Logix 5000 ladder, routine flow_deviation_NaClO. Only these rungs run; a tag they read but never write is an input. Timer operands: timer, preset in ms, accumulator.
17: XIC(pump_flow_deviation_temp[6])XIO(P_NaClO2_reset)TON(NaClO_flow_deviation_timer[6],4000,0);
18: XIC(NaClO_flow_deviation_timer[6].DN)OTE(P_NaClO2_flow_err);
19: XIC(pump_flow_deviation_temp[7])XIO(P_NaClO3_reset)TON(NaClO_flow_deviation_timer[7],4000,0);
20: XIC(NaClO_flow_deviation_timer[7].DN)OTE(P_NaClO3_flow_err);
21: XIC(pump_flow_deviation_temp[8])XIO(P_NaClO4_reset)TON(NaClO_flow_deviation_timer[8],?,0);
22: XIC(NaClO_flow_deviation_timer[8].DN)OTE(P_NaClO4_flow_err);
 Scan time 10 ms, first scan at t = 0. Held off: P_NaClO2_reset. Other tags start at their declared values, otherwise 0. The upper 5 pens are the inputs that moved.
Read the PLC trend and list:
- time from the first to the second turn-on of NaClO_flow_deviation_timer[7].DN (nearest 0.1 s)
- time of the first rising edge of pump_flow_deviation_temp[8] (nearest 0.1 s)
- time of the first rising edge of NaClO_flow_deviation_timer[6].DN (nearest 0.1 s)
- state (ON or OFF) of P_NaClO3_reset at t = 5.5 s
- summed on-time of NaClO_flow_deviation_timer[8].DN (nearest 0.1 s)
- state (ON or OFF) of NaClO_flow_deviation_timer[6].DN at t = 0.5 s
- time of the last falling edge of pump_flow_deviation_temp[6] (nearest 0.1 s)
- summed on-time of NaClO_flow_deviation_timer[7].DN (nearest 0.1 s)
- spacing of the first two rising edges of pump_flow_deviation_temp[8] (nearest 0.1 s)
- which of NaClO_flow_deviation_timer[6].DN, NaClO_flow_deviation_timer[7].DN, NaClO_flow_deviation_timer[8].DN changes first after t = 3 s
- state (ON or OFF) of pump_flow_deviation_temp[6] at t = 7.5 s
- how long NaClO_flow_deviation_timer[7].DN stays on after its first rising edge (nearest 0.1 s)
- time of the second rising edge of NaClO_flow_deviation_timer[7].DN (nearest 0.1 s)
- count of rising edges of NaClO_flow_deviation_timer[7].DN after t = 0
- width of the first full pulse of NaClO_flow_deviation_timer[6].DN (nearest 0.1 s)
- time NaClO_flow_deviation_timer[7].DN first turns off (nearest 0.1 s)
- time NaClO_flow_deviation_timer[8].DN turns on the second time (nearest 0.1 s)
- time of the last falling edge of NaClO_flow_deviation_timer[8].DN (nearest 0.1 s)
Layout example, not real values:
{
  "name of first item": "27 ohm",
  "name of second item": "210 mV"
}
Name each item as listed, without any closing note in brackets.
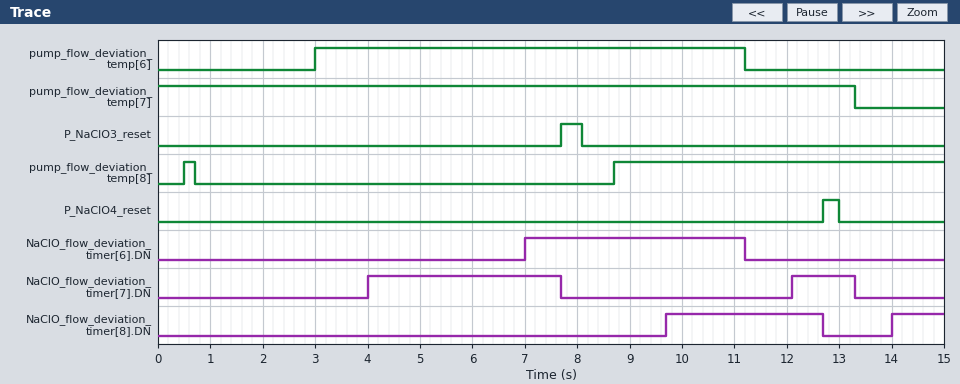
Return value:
{
  "time from the first to the second turn-on of NaClO_flow_deviation_timer[7].DN": "8.1 s",
  "time of the first rising edge of pump_flow_deviation_temp[8]": "0.5 s",
  "time of the first rising edge of NaClO_flow_deviation_timer[6].DN": "7.0 s",
  "state (ON or OFF) of P_NaClO3_reset at t = 5.5 s": "OFF",
  "summed on-time of NaClO_flow_deviation_timer[8].DN": "4.0 s",
  "state (ON or OFF) of NaClO_flow_deviation_timer[6].DN at t = 0.5 s": "OFF",
  "time of the last falling edge of pump_flow_deviation_temp[6]": "11.2 s",
  "summed on-time of NaClO_flow_deviation_timer[7].DN": "4.9 s",
  "spacing of the first two rising edges of pump_flow_deviation_temp[8]": "8.2 s",
  "which of NaClO_flow_deviation_timer[6].DN, NaClO_flow_deviation_timer[7].DN, NaClO_flow_deviation_timer[8].DN changes first after t = 3 s": "NaClO_flow_deviation_timer[7].DN",
  "state (ON or OFF) of pump_flow_deviation_temp[6] at t = 7.5 s": "ON",
  "how long NaClO_flow_deviation_timer[7].DN stays on after its first rising edge": "3.7 s",
  "time of the second rising edge of NaClO_flow_deviation_timer[7].DN": "12.1 s",
  "count of rising edges of NaClO_flow_deviation_timer[7].DN after t = 0": "2",
  "width of the first full pulse of NaClO_flow_deviation_timer[6].DN": "4.2 s",
  "time NaClO_flow_deviation_timer[7].DN first turns off": "7.7 s",
  "time NaClO_flow_deviation_timer[8].DN turns on the second time": "14.0 s",
  "time of the last falling edge of NaClO_flow_deviation_timer[8].DN": "12.7 s"
}
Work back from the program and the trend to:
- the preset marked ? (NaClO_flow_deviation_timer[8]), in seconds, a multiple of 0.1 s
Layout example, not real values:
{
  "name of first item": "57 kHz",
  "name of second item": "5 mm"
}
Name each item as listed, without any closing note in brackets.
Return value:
{
  "the preset marked ? (NaClO_flow_deviation_timer[8]), in seconds, a multiple of 0.1 s": "1.0 s"
}
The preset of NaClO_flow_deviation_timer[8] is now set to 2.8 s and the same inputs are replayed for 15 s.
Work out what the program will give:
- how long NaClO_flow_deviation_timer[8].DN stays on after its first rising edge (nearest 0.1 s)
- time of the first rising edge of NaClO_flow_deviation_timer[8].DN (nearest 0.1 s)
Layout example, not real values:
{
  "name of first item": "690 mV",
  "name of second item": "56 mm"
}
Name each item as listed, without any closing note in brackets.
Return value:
{
  "how long NaClO_flow_deviation_timer[8].DN stays on after its first rising edge": "1.2 s",
  "time of the first rising edge of NaClO_flow_deviation_timer[8].DN": "11.5 s"
}
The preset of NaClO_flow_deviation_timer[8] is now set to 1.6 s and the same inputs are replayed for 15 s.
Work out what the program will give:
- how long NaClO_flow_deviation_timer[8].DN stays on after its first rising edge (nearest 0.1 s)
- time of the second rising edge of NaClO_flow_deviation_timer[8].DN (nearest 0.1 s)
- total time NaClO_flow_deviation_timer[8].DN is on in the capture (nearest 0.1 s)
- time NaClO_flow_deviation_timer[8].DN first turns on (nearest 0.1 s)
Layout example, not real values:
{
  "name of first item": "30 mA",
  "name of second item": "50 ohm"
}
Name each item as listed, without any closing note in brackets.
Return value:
{
  "how long NaClO_flow_deviation_timer[8].DN stays on after its first rising edge": "2.4 s",
  "time of the second rising edge of NaClO_flow_deviation_timer[8].DN": "14.6 s",
  "total time NaClO_flow_deviation_timer[8].DN is on in the capture": "2.8 s",
  "time NaClO_flow_deviation_timer[8].DN first turns on": "10.3 s"
}
